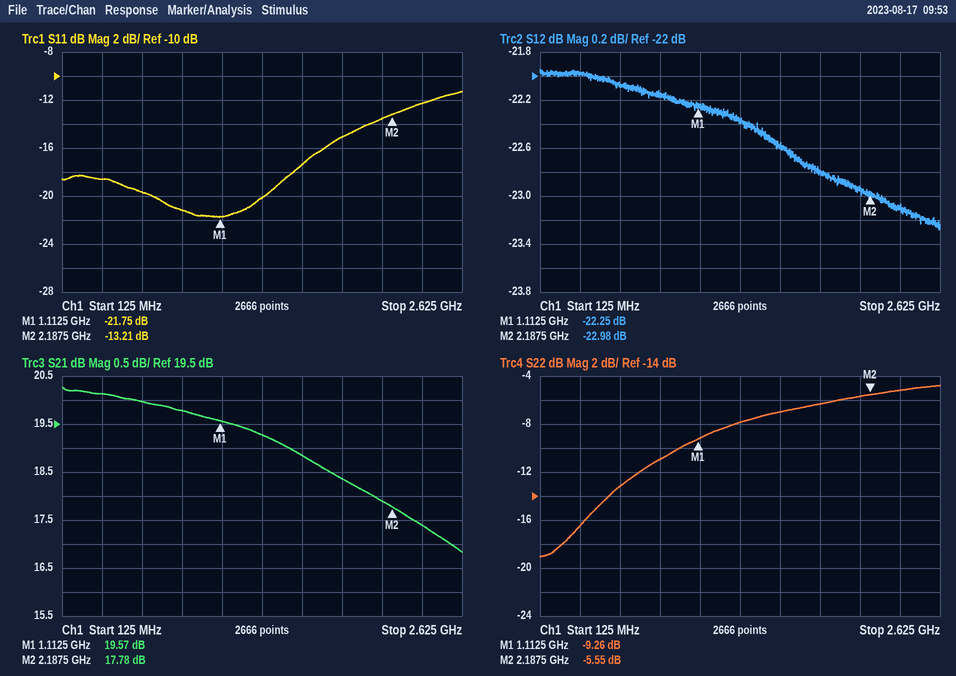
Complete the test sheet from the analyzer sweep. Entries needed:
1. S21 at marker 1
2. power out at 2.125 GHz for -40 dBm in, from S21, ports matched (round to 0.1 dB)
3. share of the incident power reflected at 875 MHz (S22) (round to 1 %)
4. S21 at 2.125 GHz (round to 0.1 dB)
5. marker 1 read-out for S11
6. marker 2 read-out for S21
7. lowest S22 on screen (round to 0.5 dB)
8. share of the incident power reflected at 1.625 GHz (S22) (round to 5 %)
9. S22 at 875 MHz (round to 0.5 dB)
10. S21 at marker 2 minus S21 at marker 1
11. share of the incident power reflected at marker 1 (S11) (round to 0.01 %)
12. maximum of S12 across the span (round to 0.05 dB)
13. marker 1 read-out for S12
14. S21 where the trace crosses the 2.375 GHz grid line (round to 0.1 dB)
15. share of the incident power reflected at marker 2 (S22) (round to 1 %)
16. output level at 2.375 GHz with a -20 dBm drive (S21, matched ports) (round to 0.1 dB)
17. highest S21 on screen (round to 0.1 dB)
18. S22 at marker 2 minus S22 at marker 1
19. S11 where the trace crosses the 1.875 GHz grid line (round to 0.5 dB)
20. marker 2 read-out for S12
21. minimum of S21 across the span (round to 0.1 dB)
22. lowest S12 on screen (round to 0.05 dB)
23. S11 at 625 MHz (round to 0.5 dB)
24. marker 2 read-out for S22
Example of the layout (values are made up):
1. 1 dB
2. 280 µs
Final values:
1. 19.57 dB
2. -22.1 dBm
3. 8 %
4. 17.9 dB
5. -21.75 dB
6. 17.78 dB
7. -19.0 dB
8. 20 %
9. -11.0 dB
10. -1.79 dB
11. 0.67 %
12. -21.95 dB
13. -22.25 dB
14. 17.4 dB
15. 28 %
16. -2.6 dBm
17. 20.3 dB
18. 3.71 dB
19. -15.0 dB
20. -22.98 dB
21. 16.8 dB
22. -23.30 dB
23. -19.5 dB
24. -5.55 dB
